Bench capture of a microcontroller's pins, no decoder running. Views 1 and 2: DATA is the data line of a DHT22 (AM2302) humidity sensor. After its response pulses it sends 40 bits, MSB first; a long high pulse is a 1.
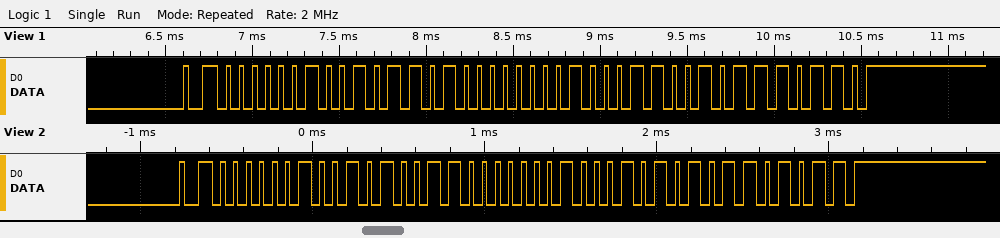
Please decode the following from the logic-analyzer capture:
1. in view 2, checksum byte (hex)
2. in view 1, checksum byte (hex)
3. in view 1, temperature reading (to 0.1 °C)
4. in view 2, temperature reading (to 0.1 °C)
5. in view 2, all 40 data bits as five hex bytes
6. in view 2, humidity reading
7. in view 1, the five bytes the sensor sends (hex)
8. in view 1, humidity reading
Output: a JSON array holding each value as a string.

["0x6B", "0x76", "28.1 °C", "27.7 °C", "02 53 01 15 6B", "59.5 %", "02 5A 01 19 76", "60.2 %"]
